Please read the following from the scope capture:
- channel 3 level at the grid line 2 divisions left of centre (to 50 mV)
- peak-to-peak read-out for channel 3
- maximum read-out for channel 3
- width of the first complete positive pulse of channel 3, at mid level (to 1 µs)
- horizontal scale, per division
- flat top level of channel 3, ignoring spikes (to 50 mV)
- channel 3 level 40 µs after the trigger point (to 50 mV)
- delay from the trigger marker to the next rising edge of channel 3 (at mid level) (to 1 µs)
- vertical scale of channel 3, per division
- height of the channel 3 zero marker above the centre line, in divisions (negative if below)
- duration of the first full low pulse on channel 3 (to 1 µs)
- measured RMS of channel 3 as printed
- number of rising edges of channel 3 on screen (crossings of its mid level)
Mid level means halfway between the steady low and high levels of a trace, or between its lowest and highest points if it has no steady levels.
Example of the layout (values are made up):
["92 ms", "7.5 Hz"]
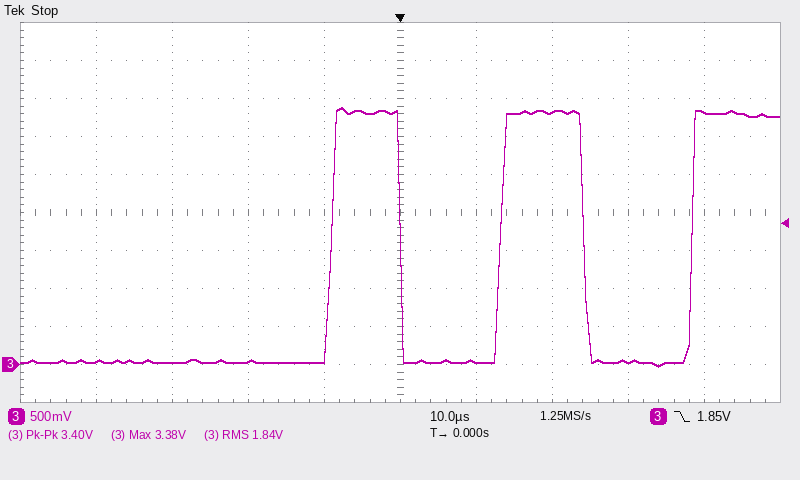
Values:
["50 mV", "3.40 V", "3.38 V", "9 µs", "10 µs", "3.30 V", "3.30 V", "13 µs", "500 mV", "-4.0 div", "13 µs", "1.84 V", "3"]
